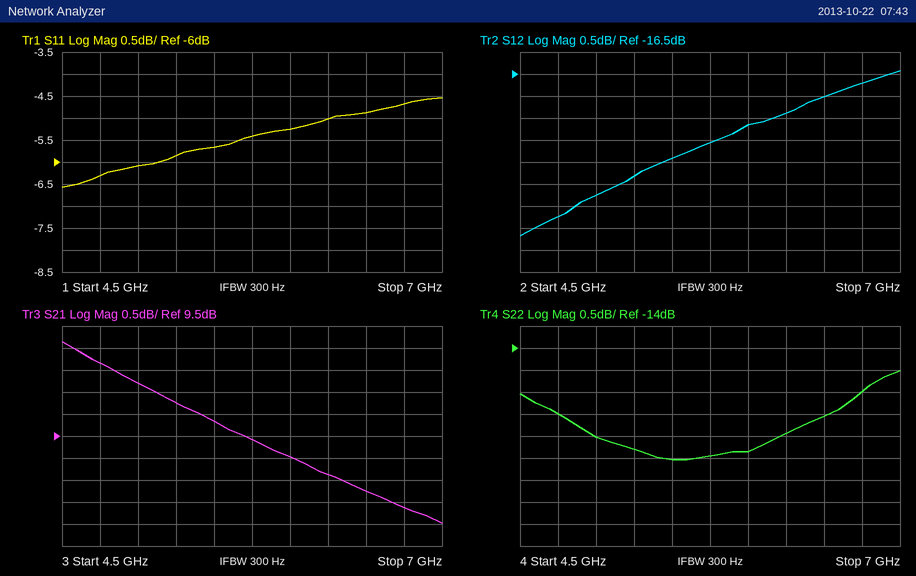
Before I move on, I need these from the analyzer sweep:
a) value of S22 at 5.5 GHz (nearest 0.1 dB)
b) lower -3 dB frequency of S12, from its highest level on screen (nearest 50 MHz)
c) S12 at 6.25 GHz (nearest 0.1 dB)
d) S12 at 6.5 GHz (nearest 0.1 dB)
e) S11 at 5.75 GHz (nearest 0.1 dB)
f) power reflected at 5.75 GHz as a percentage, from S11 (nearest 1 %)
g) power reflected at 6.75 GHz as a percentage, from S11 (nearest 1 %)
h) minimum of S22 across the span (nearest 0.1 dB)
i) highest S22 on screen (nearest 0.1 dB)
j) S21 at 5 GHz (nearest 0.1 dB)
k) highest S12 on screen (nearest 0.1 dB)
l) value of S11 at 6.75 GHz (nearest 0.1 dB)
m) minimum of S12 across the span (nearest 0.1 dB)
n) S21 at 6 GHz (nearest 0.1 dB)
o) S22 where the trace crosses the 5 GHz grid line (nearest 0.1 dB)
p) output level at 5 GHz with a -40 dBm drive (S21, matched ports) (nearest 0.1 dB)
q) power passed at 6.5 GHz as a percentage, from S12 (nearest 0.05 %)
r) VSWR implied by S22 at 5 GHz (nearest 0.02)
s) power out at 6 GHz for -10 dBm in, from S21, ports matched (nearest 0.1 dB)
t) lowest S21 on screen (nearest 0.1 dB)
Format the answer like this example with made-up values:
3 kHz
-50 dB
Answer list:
-16.5 dB
4.90 GHz
-17.4 dB
-17.0 dB
-5.4 dB
29 %
34 %
-16.5 dB
-14.5 dB
10.7 dB
-16.4 dB
-4.7 dB
-20.2 dB
9.0 dB
-16.0 dB
-29.3 dBm
2.00 %
1.38
-1.0 dBm
7.5 dB
